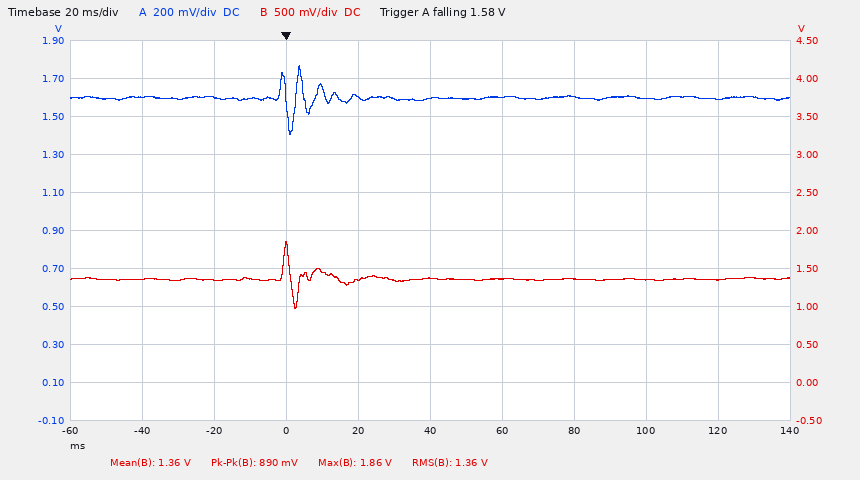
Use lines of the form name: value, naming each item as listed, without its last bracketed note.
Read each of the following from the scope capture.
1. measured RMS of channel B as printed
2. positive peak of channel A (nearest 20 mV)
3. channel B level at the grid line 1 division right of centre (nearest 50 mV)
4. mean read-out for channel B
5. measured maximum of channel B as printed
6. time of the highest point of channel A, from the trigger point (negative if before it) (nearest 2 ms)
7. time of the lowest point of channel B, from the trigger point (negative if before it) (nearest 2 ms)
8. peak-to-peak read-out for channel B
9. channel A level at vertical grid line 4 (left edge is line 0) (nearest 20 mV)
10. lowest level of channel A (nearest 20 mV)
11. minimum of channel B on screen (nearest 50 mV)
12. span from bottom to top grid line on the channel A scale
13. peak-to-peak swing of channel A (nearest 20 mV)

measured RMS of channel B as printed: 1.36 V
positive peak of channel A: 1.76 V
channel B level at the grid line 1 division right of centre: 1.35 V
mean read-out for channel B: 1.36 V
measured maximum of channel B as printed: 1.86 V
time of the highest point of channel A, from the trigger point (negative if before it): +4 ms
time of the lowest point of channel B, from the trigger point (negative if before it): +2 ms
peak-to-peak read-out for channel B: 890 mV
channel A level at vertical grid line 4 (left edge is line 0): 1.60 V
lowest level of channel A: 1.40 V
minimum of channel B on screen: 950 mV
span from bottom to top grid line on the channel A scale: 2 V
peak-to-peak swing of channel A: 360 mV
